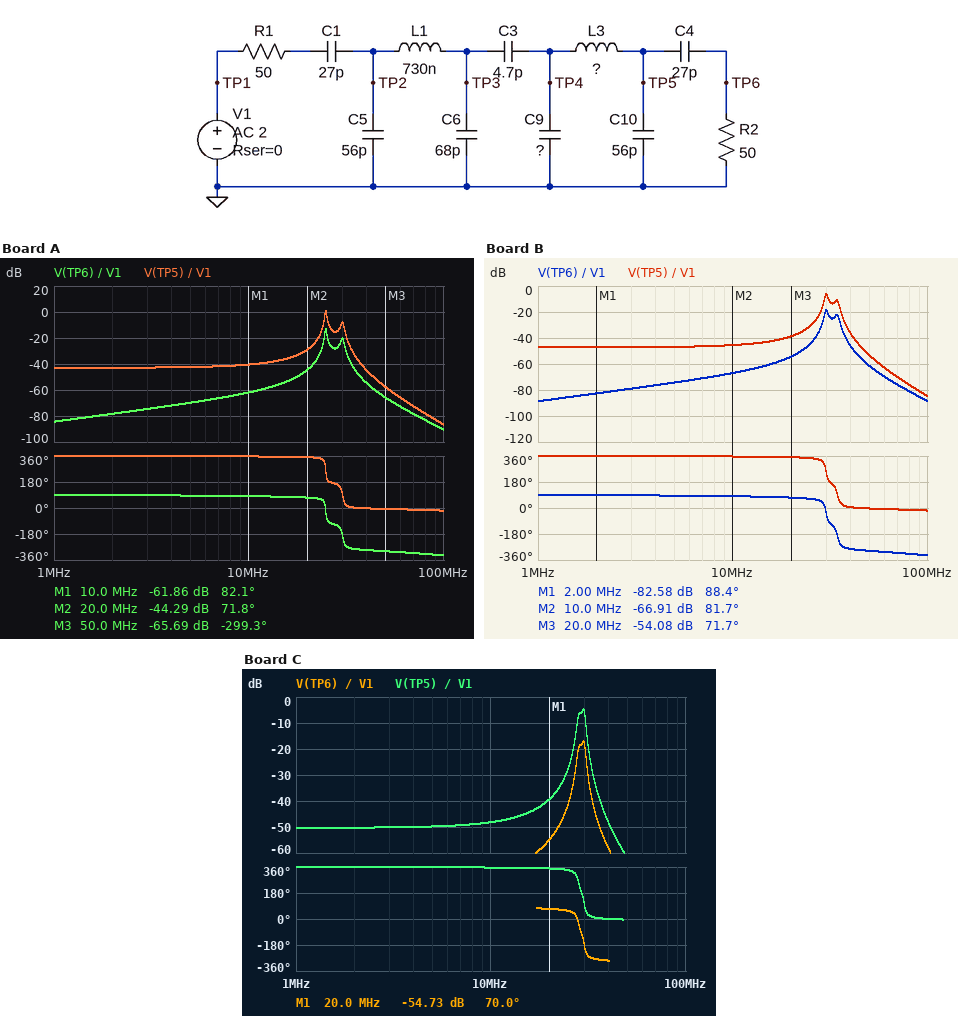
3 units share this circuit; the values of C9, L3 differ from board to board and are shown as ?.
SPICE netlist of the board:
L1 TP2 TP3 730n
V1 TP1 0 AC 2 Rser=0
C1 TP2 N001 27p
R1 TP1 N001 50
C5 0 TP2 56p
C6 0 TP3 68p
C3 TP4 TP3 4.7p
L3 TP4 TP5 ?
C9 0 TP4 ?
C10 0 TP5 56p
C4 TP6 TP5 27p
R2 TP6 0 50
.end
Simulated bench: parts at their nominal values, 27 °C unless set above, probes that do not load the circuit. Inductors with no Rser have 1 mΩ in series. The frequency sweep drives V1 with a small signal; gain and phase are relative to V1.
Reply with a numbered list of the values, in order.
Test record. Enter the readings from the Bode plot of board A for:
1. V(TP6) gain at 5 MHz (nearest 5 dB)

1. -70 dB
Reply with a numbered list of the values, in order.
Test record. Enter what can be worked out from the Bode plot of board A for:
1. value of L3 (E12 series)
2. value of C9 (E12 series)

1. 1.8 µH
2. 27 pF
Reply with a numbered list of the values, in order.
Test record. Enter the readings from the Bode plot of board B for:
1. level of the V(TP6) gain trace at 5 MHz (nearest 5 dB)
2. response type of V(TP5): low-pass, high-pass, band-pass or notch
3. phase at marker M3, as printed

1. -75 dB
2. band-pass
3. 71.7 deg
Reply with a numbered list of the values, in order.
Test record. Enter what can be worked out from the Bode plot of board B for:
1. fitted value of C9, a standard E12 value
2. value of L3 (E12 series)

1. 100 pF
2. 470 nH
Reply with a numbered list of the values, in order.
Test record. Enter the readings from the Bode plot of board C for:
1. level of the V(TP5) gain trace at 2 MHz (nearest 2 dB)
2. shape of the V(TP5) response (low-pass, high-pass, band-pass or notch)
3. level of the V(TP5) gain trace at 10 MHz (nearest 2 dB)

1. -50 dB
2. band-pass
3. -48 dB
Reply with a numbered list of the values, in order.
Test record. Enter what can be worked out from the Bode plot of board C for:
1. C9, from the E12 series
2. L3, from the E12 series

1. 180 pF
2. 560 nH
